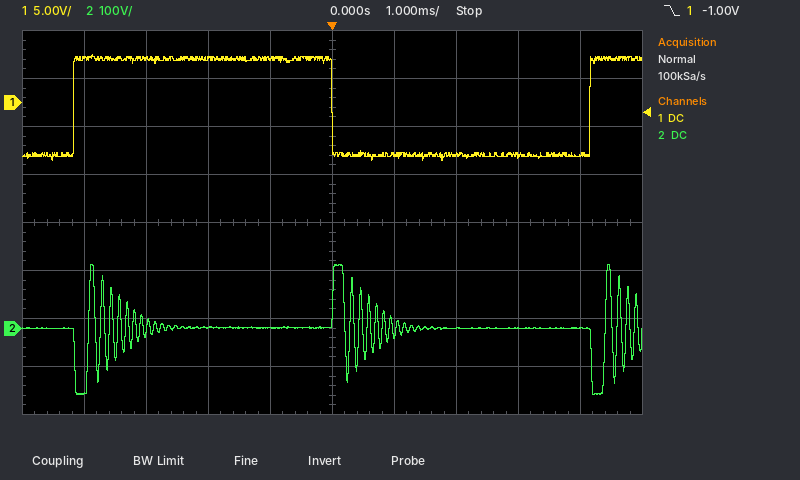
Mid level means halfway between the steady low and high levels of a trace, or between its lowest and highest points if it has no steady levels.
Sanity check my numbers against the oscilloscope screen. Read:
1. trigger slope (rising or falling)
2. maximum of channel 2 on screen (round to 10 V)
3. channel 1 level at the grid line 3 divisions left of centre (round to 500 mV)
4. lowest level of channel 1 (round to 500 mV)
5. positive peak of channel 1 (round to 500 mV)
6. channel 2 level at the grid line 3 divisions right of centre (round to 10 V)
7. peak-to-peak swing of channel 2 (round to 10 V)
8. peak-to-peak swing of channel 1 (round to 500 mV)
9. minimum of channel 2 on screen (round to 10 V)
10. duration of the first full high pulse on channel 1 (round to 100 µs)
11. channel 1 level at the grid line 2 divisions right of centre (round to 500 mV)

falling
130 V
4.5 V
-6.0 V
5.0 V
0 V
270 V
11.0 V
-140 V
4.2 ms
-5.5 V
